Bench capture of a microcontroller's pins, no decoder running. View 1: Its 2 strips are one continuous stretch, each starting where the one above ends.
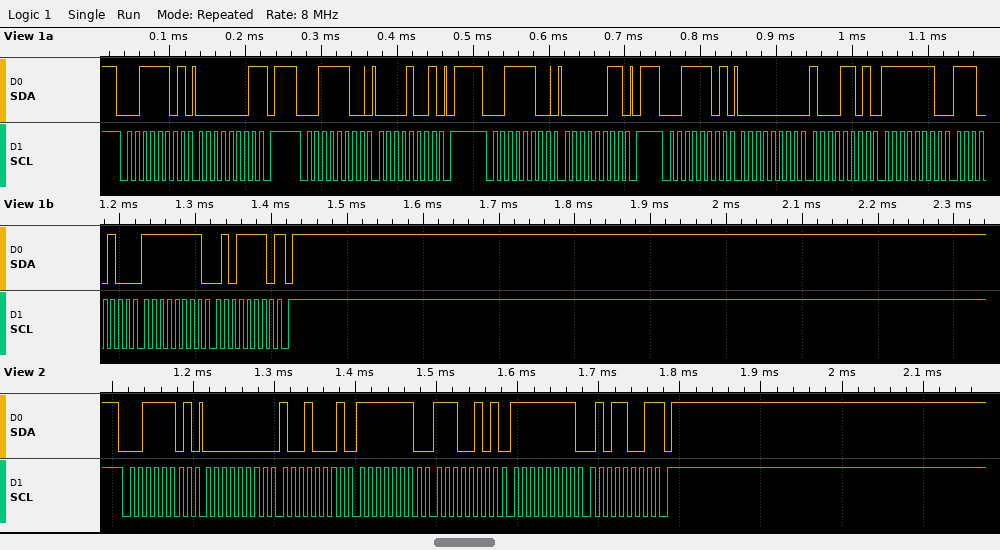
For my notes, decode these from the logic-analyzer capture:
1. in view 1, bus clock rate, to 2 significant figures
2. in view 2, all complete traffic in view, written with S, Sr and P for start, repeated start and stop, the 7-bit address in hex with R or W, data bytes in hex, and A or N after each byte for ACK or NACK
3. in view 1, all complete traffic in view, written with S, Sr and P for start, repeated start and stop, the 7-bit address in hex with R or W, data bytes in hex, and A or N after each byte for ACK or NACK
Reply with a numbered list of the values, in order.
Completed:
1. 100 kHz
2. S 1ER A 00 A 91 A FE A E5 A FF A 59 N P
3. S 1ER A 01 N P S 1EW A 09 A P S 1EW A 03 A P S 1ER A 00 A 8D A FE A E4 A FF A 5E N P
